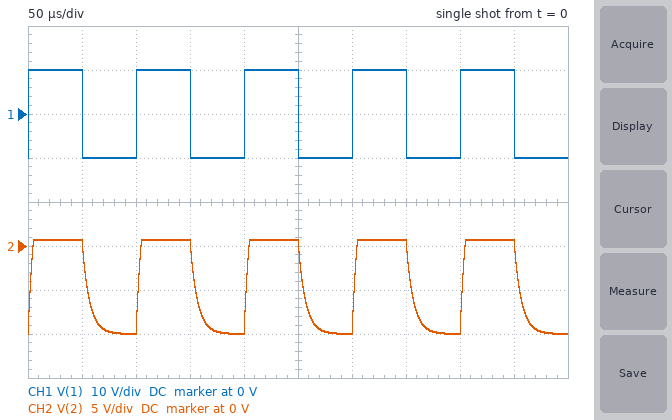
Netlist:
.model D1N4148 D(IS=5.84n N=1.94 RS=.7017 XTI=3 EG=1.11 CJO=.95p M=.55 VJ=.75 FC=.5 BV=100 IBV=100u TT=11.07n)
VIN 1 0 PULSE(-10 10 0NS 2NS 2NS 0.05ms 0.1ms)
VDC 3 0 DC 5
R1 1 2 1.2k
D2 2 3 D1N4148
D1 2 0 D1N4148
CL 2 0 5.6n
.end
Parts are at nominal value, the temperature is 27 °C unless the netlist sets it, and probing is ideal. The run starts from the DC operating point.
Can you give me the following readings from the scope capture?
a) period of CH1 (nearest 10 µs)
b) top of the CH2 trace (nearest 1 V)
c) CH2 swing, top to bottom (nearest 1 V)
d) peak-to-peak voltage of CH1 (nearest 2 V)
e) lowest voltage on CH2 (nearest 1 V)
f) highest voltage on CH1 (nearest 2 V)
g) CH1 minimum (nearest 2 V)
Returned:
100 µs
1 V
11 V
20 V
-10 V
10 V
-10 V
